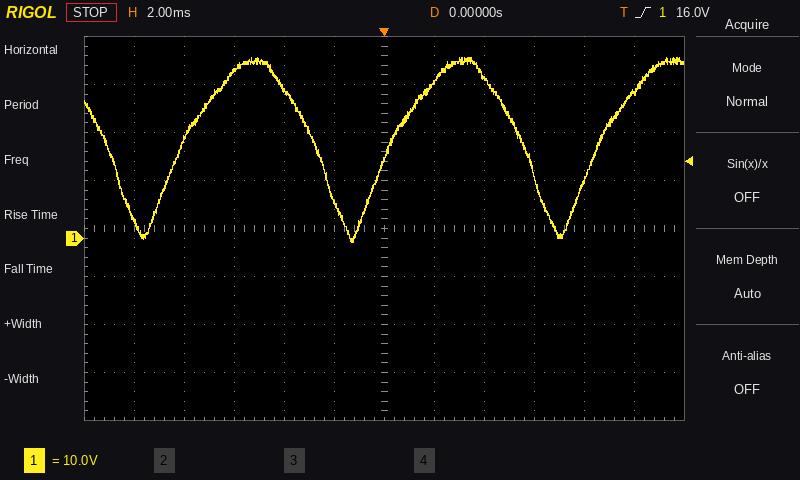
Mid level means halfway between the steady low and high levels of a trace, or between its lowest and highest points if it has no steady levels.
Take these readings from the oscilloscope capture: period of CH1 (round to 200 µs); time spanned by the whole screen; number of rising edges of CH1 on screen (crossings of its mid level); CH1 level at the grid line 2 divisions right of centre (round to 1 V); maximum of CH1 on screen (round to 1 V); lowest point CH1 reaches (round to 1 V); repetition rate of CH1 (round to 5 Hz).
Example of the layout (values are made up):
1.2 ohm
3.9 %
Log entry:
8.4 ms
24 ms
3
34 V
38 V
-1 V
120 Hz
